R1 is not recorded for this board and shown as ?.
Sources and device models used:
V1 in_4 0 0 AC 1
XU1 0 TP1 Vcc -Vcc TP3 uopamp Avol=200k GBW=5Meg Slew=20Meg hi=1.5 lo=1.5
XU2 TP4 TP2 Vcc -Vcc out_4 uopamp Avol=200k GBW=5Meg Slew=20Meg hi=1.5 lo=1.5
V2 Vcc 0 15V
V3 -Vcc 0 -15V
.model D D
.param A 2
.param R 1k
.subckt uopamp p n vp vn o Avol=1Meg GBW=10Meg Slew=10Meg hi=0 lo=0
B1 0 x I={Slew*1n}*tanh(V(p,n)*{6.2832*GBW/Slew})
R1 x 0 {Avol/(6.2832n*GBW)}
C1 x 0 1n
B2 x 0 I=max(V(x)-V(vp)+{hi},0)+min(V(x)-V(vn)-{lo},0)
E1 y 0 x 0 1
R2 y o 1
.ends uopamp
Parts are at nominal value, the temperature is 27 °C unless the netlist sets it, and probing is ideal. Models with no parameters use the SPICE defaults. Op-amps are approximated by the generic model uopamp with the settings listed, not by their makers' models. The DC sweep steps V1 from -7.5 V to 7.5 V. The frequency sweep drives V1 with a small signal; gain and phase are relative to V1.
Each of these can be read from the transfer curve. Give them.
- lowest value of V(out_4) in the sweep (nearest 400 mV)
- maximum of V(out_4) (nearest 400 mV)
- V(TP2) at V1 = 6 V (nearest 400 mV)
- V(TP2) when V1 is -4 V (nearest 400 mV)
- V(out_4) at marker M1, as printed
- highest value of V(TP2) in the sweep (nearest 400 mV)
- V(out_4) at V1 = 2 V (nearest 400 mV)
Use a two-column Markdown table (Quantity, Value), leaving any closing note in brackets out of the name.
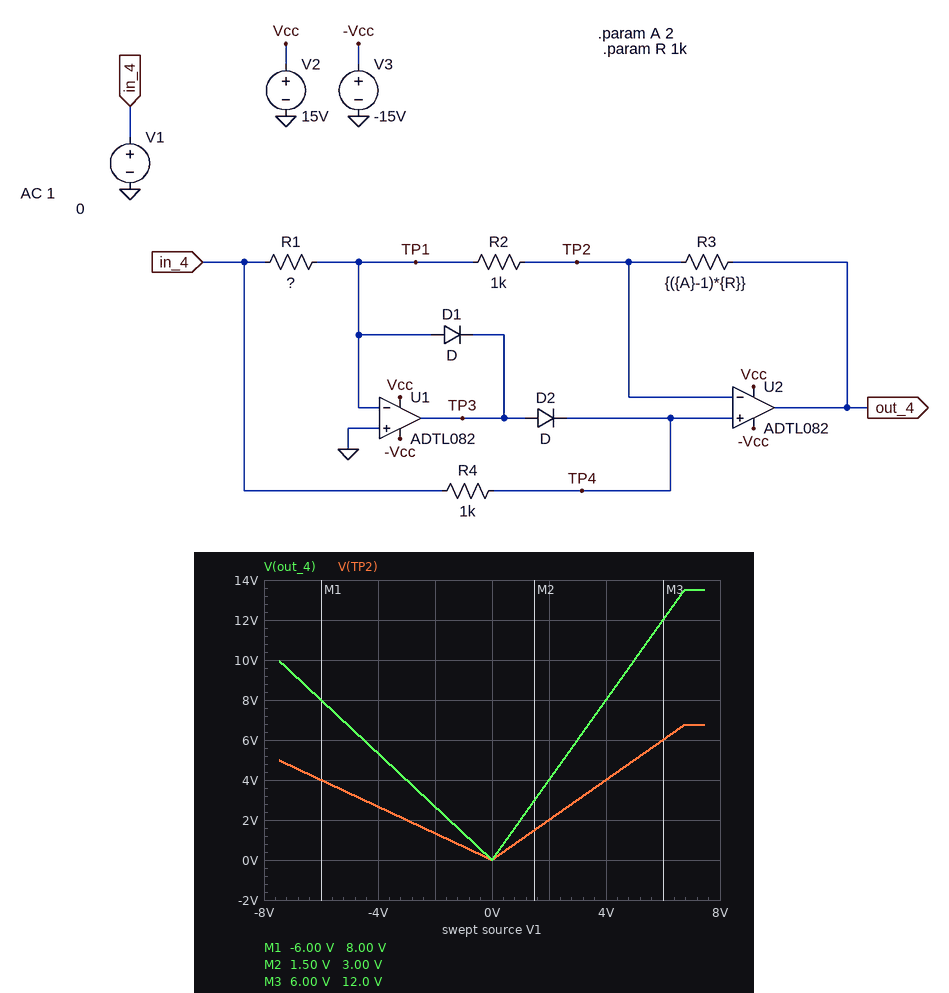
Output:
| Quantity | Value |
|---|---|
| lowest value of V(out_4) in the sweep | 0 V |
| maximum of V(out_4) | 13.6 V |
| V(TP2) at V1 = 6 V | 6.0 V |
| V(TP2) when V1 is -4 V | 2.8 V |
| V(out_4) at marker M1, as printed | 8.00 V |
| highest value of V(TP2) in the sweep | 6.8 V |
| V(out_4) at V1 = 2 V | 4.0 V |
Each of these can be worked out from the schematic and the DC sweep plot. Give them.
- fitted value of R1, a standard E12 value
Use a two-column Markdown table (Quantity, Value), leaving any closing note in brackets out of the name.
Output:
| Quantity | Value |
|---|---|
| fitted value of R1, a standard E12 value | 1.5 kΩ |
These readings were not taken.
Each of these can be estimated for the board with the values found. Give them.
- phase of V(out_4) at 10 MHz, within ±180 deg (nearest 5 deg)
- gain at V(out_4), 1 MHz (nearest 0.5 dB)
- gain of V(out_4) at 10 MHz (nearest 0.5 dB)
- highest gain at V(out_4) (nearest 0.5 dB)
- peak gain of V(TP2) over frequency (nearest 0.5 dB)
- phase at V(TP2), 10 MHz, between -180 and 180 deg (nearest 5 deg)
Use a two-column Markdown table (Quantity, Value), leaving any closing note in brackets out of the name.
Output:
| Quantity | Value |
|---|---|
| phase of V(out_4) at 10 MHz, within ±180 deg | -70 deg |
| gain at V(out_4), 1 MHz | -0.5 dB |
| gain of V(out_4) at 10 MHz | -9.5 dB |
| highest gain at V(out_4) | 0 dB |
| peak gain of V(TP2) over frequency | 0 dB |
| phase at V(TP2), 10 MHz, between -180 and 180 deg | -30 deg |
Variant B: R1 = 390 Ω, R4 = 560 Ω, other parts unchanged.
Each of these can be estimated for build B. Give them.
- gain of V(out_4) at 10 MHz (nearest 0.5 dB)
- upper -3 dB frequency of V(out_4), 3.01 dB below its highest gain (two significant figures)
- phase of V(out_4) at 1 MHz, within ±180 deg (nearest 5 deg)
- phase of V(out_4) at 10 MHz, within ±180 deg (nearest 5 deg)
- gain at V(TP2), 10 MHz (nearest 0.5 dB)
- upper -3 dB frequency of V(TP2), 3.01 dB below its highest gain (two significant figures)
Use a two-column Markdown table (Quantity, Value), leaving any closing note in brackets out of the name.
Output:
| Quantity | Value |
|---|---|
| gain of V(out_4) at 10 MHz | -11.0 dB |
| upper -3 dB frequency of V(out_4), 3.01 dB below its highest gain | 2.9 MHz |
| phase of V(out_4) at 1 MHz, within ±180 deg | -20 deg |
| phase of V(out_4) at 10 MHz, within ±180 deg | -75 deg |
| gain at V(TP2), 10 MHz | -6.0 dB |
| upper -3 dB frequency of V(TP2), 3.01 dB below its highest gain | 3.6 MHz |
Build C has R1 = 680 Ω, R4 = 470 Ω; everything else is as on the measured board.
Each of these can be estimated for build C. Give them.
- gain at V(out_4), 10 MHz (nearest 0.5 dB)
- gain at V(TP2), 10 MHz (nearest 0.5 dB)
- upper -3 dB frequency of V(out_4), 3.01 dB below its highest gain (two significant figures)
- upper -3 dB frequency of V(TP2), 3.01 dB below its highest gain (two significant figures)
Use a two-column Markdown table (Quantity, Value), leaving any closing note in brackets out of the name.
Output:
| Quantity | Value |
|---|---|
| gain at V(out_4), 10 MHz | -10.5 dB |
| gain at V(TP2), 10 MHz | -6.5 dB |
| upper -3 dB frequency of V(out_4), 3.01 dB below its highest gain | 3.1 MHz |
| upper -3 dB frequency of V(TP2), 3.01 dB below its highest gain | 3.7 MHz |
